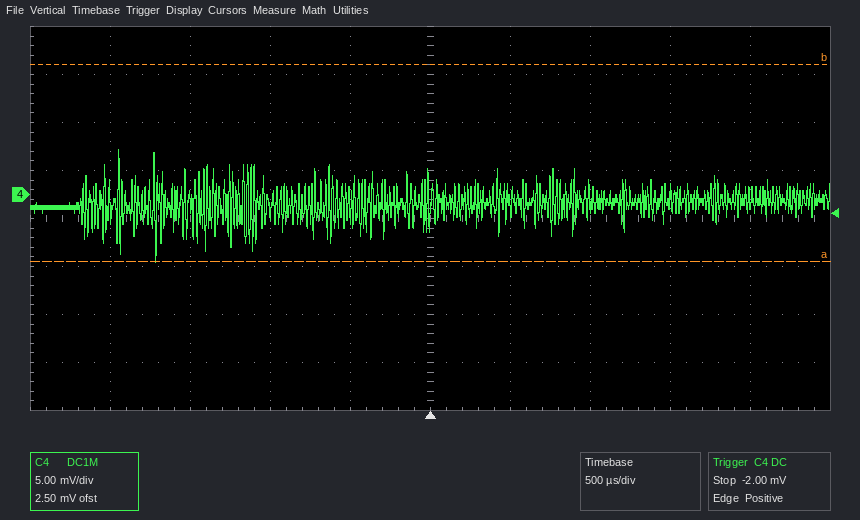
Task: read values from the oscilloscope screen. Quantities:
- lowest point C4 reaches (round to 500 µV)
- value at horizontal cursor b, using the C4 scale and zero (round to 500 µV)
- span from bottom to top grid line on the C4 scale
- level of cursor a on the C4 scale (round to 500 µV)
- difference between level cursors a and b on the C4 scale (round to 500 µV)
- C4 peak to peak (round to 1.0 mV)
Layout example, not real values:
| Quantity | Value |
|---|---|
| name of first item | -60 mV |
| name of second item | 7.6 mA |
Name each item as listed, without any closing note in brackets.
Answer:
| Quantity | Value |
|---|---|
| lowest point C4 reaches | -7.0 mV |
| value at horizontal cursor b, using the C4 scale and zero | 13.5 mV |
| span from bottom to top grid line on the C4 scale | 40 mV |
| level of cursor a on the C4 scale | -7.0 mV |
| difference between level cursors a and b on the C4 scale | 20.5 mV |
| C4 peak to peak | 12.0 mV |
